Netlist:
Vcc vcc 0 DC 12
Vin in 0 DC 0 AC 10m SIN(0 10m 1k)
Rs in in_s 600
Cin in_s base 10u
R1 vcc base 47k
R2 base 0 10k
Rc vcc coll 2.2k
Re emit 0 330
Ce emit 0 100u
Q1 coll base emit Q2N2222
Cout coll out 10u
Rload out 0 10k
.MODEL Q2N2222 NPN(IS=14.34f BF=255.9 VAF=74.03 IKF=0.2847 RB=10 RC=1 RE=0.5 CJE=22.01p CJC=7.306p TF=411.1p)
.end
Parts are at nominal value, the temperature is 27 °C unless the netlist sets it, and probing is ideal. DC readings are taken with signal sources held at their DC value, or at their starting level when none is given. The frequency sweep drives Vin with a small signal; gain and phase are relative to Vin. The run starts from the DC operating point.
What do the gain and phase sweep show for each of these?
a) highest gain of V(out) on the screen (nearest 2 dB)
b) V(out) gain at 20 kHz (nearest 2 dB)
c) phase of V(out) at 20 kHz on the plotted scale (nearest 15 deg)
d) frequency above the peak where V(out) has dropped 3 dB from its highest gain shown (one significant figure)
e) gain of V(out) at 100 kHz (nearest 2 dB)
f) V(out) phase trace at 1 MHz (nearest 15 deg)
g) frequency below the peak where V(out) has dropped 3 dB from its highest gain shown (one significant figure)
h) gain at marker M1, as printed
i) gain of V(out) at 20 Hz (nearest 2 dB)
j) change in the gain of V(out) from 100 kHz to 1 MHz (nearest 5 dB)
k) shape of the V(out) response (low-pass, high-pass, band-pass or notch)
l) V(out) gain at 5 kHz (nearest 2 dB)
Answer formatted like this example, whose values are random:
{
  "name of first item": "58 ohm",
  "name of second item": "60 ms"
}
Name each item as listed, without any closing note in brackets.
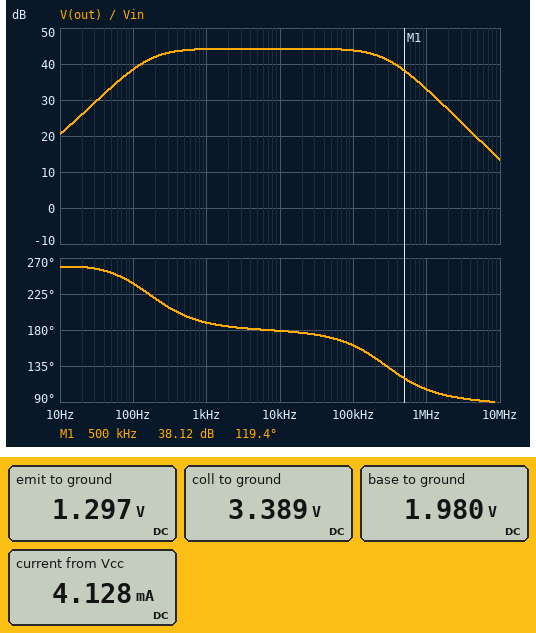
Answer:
{
  "highest gain of V(out) on the screen": "44 dB",
  "V(out) gain at 20 kHz": "44 dB",
  "phase of V(out) at 20 kHz on the plotted scale": "180 deg",
  "frequency above the peak where V(out) has dropped 3 dB from its highest gain shown": "300 kHz",
  "gain of V(out) at 100 kHz": "44 dB",
  "V(out) phase trace at 1 MHz": "105 deg",
  "frequency below the peak where V(out) has dropped 3 dB from its highest gain shown": "200 Hz",
  "gain at marker M1, as printed": "38.12 dB",
  "gain of V(out) at 20 Hz": "26 dB",
  "change in the gain of V(out) from 100 kHz to 1 MHz": "-10 dB",
  "shape of the V(out) response": "band-pass",
  "V(out) gain at 5 kHz": "44 dB"
}
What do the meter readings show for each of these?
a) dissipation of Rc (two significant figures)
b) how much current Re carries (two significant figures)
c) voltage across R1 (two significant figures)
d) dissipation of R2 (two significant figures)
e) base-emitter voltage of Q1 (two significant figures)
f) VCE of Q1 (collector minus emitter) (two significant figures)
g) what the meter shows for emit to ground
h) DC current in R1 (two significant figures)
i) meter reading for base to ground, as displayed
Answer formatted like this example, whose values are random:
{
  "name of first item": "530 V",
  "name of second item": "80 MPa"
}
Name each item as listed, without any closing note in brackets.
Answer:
{
  "dissipation of Rc": "34 mW",
  "how much current Re carries": "3.9 mA",
  "voltage across R1": "10 V",
  "dissipation of R2": "390 µW",
  "base-emitter voltage of Q1": "680 mV",
  "VCE of Q1 (collector minus emitter)": "2.1 V",
  "what the meter shows for emit to ground": "1.297 V",
  "DC current in R1": "210 µA",
  "meter reading for base to ground, as displayed": "1.980 V"
}
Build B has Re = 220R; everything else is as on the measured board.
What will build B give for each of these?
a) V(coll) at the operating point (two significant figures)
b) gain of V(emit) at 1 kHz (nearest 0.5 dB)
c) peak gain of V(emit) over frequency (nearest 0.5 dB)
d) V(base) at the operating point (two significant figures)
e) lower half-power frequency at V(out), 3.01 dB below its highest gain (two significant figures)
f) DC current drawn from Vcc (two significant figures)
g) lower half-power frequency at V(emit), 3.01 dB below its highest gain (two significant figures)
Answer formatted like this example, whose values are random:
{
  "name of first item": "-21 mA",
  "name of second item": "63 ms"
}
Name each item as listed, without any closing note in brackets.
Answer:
{
  "V(coll) at the operating point": "1.2 V",
  "gain of V(emit) at 1 kHz": "-47.5 dB",
  "peak gain of V(emit) over frequency": "-19.0 dB",
  "V(base) at the operating point": "1.8 V",
  "lower half-power frequency at V(out), 3.01 dB below its highest gain": "32 Hz",
  "DC current drawn from Vcc": "5.1 mA",
  "lower half-power frequency at V(emit), 3.01 dB below its highest gain": "5.0 Hz"
}
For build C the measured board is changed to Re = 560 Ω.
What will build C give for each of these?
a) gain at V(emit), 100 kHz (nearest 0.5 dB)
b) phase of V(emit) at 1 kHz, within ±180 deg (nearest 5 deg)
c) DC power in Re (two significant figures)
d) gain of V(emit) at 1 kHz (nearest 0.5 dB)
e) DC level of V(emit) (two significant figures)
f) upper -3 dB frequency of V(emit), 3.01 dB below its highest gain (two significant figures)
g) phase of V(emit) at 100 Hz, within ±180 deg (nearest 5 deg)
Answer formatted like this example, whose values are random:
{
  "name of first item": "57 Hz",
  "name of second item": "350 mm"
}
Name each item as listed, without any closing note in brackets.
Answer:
{
  "gain at V(emit), 100 kHz": "-59.5 dB",
  "phase of V(emit) at 1 kHz, within ±180 deg": "-85 deg",
  "DC power in Re": "3.3 mW",
  "gain of V(emit) at 1 kHz": "-19.5 dB",
  "DC level of V(emit)": "1.4 V",
  "upper -3 dB frequency of V(emit), 3.01 dB below its highest gain": "120 Hz",
  "phase of V(emit) at 100 Hz, within ±180 deg": "-40 deg"
}
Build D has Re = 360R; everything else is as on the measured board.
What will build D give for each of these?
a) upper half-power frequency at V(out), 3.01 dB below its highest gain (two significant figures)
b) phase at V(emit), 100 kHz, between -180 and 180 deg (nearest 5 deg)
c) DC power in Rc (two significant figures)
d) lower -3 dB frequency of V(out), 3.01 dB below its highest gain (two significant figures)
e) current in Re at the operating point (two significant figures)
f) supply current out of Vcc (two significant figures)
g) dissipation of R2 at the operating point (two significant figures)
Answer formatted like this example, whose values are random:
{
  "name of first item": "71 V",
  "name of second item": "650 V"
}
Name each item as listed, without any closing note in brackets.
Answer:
{
  "upper half-power frequency at V(out), 3.01 dB below its highest gain": "320 kHz",
  "phase at V(emit), 100 kHz, between -180 and 180 deg": "-105 deg",
  "DC power in Rc": "29 mW",
  "lower -3 dB frequency of V(out), 3.01 dB below its highest gain": "160 Hz",
  "current in Re at the operating point": "3.6 mA",
  "supply current out of Vcc": "3.8 mA",
  "dissipation of R2 at the operating point": "400 µW"
}
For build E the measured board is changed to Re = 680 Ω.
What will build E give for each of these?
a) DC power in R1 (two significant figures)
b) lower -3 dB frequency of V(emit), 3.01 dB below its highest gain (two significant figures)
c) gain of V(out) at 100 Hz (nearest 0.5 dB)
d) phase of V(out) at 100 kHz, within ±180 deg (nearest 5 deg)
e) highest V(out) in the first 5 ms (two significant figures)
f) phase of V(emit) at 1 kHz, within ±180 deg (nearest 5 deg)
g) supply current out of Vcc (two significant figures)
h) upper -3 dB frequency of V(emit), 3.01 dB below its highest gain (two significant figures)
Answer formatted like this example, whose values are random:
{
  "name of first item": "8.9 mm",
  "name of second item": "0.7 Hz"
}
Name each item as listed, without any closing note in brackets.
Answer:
{
  "DC power in R1": "2.1 mW",
  "lower -3 dB frequency of V(emit), 3.01 dB below its highest gain": "1.8 Hz",
  "gain of V(out) at 100 Hz": "37.0 dB",
  "phase of V(out) at 100 kHz, within ±180 deg": "170 deg",
  "highest V(out) in the first 5 ms": "990 mV",
  "phase of V(emit) at 1 kHz, within ±180 deg": "-85 deg",
  "supply current out of Vcc": "2.2 mA",
  "upper -3 dB frequency of V(emit), 3.01 dB below its highest gain": "110 Hz"
}
